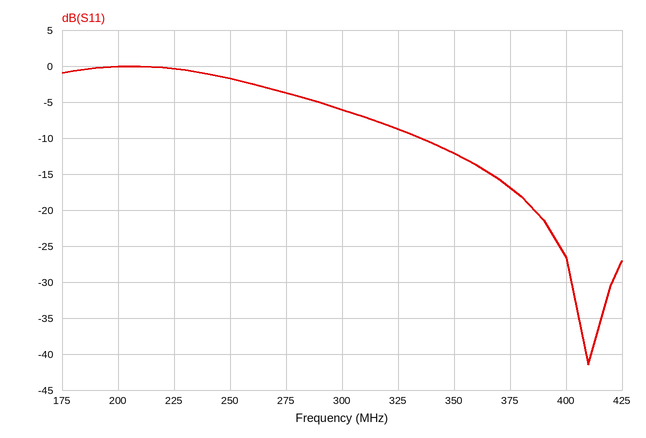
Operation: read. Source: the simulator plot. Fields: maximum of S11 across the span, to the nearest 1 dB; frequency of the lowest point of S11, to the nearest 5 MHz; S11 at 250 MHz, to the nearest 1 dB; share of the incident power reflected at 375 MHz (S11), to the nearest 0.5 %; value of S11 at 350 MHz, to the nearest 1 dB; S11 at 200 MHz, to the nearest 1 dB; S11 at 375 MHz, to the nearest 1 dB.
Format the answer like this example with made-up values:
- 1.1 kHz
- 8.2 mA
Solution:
- 0 dB
- 410 MHz
- -2 dB
- 2.0 %
- -12 dB
- 0 dB
- -17 dB
